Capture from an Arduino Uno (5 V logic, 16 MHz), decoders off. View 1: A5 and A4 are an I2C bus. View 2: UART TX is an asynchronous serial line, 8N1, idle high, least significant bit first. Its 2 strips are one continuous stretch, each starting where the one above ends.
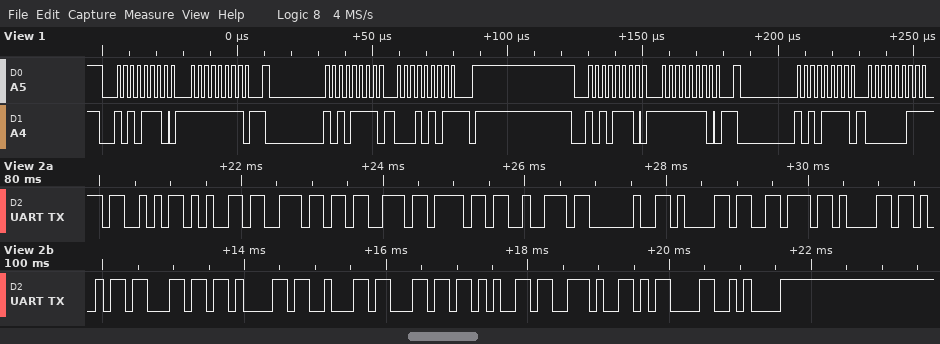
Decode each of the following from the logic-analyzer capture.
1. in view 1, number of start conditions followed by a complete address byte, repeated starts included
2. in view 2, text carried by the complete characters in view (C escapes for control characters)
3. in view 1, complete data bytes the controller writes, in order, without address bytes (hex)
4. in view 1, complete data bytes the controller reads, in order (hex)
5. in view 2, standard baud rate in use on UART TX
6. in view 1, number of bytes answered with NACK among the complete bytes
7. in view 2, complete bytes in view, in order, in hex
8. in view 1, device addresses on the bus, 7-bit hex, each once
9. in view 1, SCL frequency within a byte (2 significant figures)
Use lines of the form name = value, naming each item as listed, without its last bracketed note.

in view 1, number of start conditions followed by a complete address byte, repeated starts included = 4
in view 2, text carried by the complete characters in view = "Sensor available.\r\n"
in view 1, complete data bytes the controller writes, in order, without address bytes = FF FE
in view 1, complete data bytes the controller reads, in order = 15 03
in view 2, standard baud rate in use on UART TX = 9600 baud
in view 1, number of bytes answered with NACK among the complete bytes = 2
in view 2, complete bytes in view, in order, in hex = 0x53 0x65 0x6E 0x73 0x6F 0x72 0x20 0x61 0x76 0x61 0x69 0x6C 0x61 0x62 0x6C 0x65 0x2E 0x0D 0x0A
in view 1, device addresses on the bus, 7-bit hex, each once = 0x57
in view 1, SCL frequency within a byte = 400 kHz
